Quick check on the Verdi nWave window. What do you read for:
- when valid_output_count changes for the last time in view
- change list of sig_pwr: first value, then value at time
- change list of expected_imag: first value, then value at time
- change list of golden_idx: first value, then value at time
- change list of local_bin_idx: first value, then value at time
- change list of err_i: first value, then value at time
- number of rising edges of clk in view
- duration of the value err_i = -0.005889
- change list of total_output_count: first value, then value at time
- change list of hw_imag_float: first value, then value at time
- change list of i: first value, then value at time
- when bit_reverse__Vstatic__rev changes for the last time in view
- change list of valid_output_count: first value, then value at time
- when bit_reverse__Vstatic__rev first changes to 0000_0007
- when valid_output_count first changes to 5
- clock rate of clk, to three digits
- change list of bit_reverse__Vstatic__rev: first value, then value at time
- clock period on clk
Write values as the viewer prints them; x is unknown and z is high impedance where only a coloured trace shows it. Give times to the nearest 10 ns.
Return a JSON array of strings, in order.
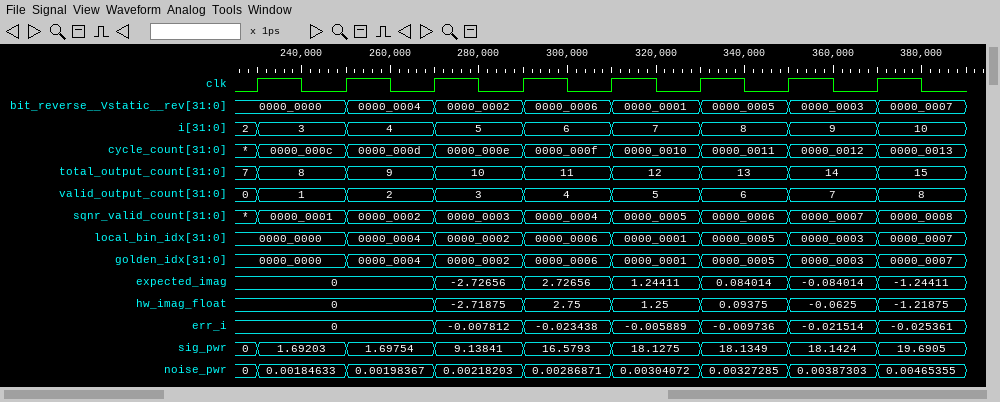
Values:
["370 ns", "0, 1.69203 at 230 ns, 1.69754 at 250 ns, 9.13841 at 270 ns, 16.5793 at 290 ns, 18.1275 at 310 ns, 18.1349 at 330 ns, 18.1424 at 350 ns, 19.6905 at 370 ns", "0, -2.72656 at 270 ns, 2.72656 at 290 ns, 1.24411 at 310 ns, 0.084014 at 330 ns, -0.084014 at 350 ns, -1.24411 at 370 ns", "0000_0000, 0000_0004 at 250 ns, 0000_0002 at 270 ns, 0000_0006 at 290 ns, 0000_0001 at 310 ns, 0000_0005 at 330 ns, 0000_0003 at 350 ns, 0000_0007 at 370 ns", "0000_0000, 0000_0004 at 250 ns, 0000_0002 at 270 ns, 0000_0006 at 290 ns, 0000_0001 at 310 ns, 0000_0005 at 330 ns, 0000_0003 at 350 ns, 0000_0007 at 370 ns", "0, -0.007812 at 270 ns, -0.023438 at 290 ns, -0.005889 at 310 ns, -0.009736 at 330 ns, -0.021514 at 350 ns, -0.025361 at 370 ns", "8", "20 ns", "7, 8 at 230 ns, 9 at 250 ns, 10 at 270 ns, 11 at 290 ns, 12 at 310 ns, 13 at 330 ns, 14 at 350 ns, 15 at 370 ns", "0, -2.71875 at 270 ns, 2.75 at 290 ns, 1.25 at 310 ns, 0.09375 at 330 ns, -0.0625 at 350 ns, -1.21875 at 370 ns", "2, 3 at 230 ns, 4 at 250 ns, 5 at 270 ns, 6 at 290 ns, 7 at 310 ns, 8 at 330 ns, 9 at 350 ns, 10 at 370 ns", "370 ns", "0, 1 at 230 ns, 2 at 250 ns, 3 at 270 ns, 4 at 290 ns, 5 at 310 ns, 6 at 330 ns, 7 at 350 ns, 8 at 370 ns", "370 ns", "310 ns", "50.0 MHz", "0000_0000, 0000_0004 at 250 ns, 0000_0002 at 270 ns, 0000_0006 at 290 ns, 0000_0001 at 310 ns, 0000_0005 at 330 ns, 0000_0003 at 350 ns, 0000_0007 at 370 ns", "20 ns"]
